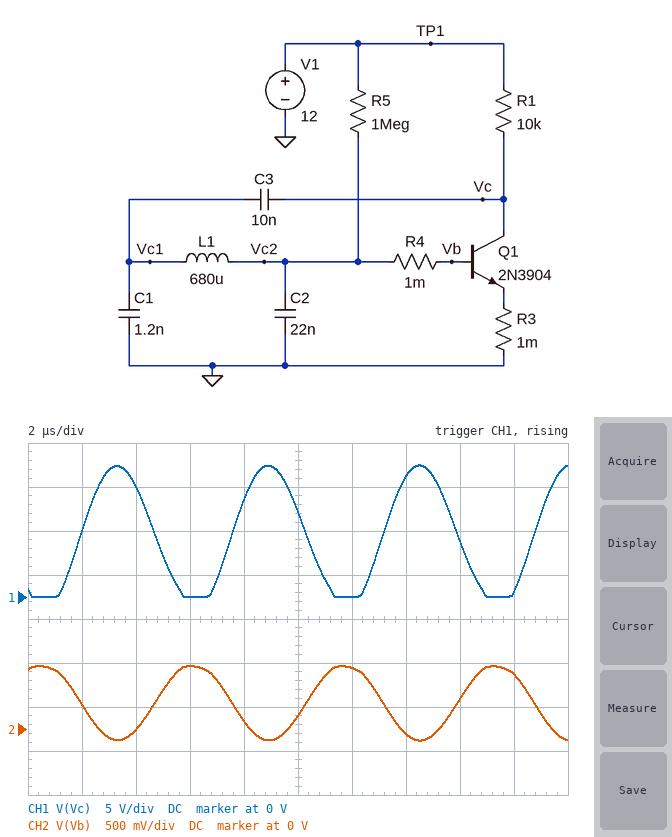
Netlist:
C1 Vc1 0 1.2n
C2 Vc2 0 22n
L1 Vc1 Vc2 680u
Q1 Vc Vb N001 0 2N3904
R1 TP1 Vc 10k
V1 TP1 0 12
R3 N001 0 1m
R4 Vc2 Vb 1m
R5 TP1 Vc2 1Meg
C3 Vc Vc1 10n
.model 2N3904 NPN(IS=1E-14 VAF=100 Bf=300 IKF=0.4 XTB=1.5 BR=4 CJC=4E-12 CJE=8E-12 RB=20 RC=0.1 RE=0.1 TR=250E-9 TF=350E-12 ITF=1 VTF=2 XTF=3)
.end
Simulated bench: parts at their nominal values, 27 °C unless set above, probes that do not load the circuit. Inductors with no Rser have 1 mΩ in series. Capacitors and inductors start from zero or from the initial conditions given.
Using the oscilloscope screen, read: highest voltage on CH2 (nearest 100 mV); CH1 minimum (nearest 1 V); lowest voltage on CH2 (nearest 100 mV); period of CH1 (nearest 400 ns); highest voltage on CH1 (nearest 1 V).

700 mV
0 V
-100 mV
5.6 µs
15 V
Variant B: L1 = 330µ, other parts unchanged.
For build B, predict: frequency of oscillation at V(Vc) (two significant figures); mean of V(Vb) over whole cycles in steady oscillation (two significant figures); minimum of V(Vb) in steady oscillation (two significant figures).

260 kHz
290 mV
-150 mV
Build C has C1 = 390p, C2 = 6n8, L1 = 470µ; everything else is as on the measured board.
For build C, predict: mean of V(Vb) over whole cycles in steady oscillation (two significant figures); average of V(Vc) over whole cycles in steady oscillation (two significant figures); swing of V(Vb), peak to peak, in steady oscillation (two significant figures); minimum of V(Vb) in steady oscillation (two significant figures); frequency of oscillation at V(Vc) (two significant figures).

290 mV
6.8 V
900 mV
-180 mV
370 kHz
